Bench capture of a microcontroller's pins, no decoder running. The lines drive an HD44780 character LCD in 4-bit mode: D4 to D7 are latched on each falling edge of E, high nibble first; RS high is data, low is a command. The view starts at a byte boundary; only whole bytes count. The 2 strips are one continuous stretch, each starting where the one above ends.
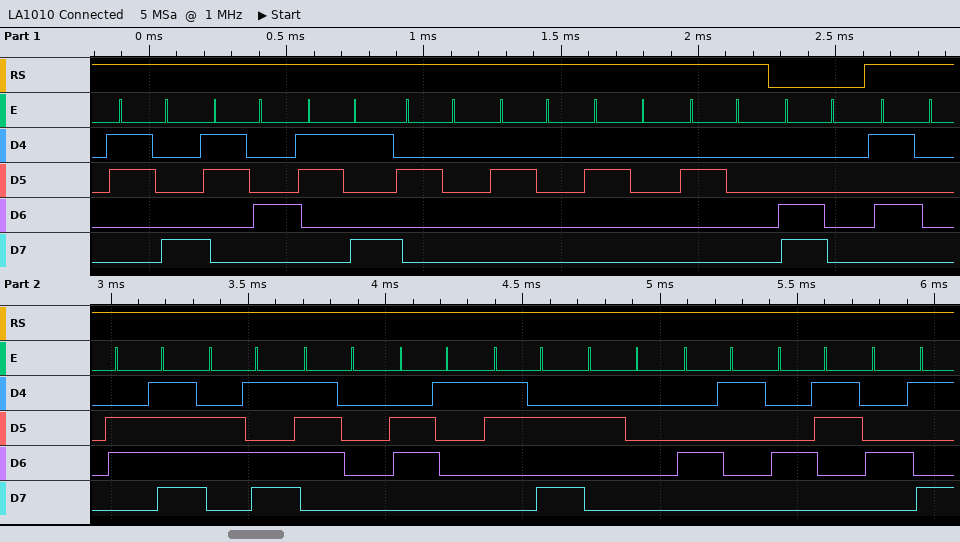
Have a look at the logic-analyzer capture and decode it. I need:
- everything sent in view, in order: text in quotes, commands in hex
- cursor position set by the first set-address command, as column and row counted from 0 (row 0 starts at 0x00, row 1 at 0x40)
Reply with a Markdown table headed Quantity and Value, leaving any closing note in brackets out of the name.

| Quantity | Value |
|---|---|
| everything sent in view, in order: text in quotes, commands in hex | "849    " 0xC0 "Pompa: ACI" |
| cursor position set by the first set-address command, as column and row counted from 0 | column 0, row 1 |
